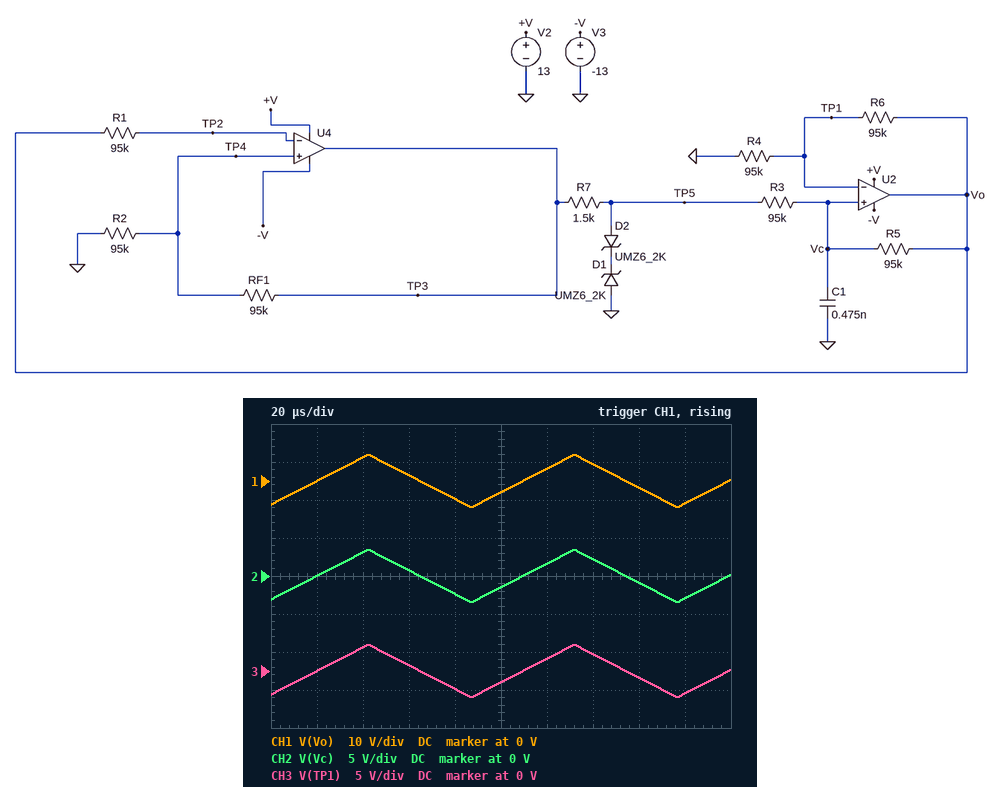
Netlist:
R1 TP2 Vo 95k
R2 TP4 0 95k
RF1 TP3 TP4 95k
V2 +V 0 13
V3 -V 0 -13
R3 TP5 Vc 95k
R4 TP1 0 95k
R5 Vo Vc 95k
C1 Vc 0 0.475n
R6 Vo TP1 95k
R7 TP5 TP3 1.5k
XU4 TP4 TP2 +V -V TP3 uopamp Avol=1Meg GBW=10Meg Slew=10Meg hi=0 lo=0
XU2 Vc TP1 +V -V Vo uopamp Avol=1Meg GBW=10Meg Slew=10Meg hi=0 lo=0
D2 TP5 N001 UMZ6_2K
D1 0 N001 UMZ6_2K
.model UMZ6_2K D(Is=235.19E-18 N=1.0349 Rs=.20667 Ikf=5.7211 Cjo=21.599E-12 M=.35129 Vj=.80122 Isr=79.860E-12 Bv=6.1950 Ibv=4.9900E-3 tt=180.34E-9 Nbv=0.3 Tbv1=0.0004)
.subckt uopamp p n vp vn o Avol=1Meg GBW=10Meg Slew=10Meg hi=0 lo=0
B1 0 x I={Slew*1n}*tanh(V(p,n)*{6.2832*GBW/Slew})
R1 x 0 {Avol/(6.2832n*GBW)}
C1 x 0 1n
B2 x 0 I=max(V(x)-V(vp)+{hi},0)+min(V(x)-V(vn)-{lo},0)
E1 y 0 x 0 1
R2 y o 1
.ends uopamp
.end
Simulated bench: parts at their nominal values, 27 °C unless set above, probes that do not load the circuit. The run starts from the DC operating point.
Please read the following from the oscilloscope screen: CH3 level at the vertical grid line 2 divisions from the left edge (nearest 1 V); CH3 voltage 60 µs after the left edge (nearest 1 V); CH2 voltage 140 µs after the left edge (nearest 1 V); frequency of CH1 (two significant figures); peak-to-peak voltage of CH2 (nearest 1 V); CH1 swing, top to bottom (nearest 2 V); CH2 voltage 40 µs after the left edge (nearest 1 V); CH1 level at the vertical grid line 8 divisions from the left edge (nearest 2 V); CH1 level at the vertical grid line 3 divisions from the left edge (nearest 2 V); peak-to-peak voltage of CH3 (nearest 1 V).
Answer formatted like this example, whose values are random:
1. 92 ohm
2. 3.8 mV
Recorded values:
1. 3 V
2. 1 V
3. 2 V
4. 11 kHz
5. 7 V
6. 14 V
7. 3 V
8. -2 V
9. 2 V
10. 7 V
